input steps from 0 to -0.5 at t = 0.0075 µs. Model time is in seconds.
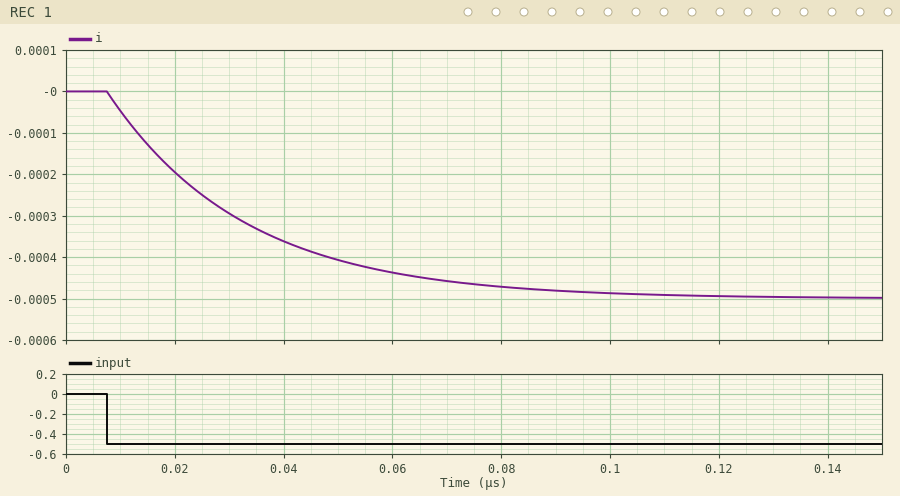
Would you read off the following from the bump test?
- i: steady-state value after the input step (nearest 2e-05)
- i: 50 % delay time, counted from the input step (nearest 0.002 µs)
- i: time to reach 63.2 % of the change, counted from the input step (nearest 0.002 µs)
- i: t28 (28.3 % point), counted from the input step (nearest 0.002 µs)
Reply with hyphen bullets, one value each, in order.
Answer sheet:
- -0.00050
- 0.018 µs
- 0.026 µs
- 0.008 µs
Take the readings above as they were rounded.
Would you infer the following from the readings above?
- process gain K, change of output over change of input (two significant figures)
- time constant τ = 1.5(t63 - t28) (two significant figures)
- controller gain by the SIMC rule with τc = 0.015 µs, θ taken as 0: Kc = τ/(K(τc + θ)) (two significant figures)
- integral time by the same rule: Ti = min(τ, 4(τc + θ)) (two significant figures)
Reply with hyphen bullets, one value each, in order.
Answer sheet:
- 0.0010
- 0.027 µs
- 1800
- 0.027 µs
